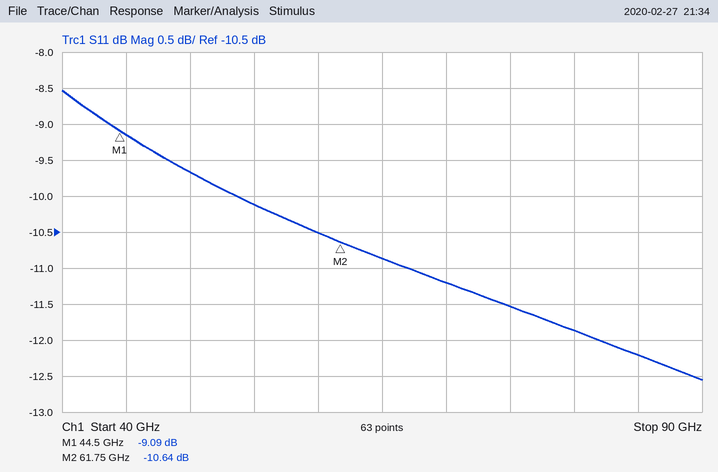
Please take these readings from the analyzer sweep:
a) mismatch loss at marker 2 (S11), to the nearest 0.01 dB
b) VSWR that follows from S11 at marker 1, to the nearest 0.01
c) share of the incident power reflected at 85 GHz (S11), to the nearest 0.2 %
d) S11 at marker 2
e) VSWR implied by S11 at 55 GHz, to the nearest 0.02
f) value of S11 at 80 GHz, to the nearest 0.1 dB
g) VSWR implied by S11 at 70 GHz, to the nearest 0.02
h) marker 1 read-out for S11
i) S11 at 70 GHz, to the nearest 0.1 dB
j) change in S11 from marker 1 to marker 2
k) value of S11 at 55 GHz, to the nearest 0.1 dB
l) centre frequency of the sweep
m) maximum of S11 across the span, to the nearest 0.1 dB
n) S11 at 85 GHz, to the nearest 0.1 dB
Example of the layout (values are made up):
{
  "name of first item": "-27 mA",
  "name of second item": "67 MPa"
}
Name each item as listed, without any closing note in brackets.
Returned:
{
  "mismatch loss at marker 2 (S11), to the nearest 0.01 dB": "0.39 dB",
  "VSWR that follows from S11 at marker 1, to the nearest 0.01": "2.08",
  "share of the incident power reflected at 85 GHz (S11), to the nearest 0.2 %": "6.0 %",
  "S11 at marker 2": "-10.64 dB",
  "VSWR implied by S11 at 55 GHz, to the nearest 0.02": "1.90",
  "value of S11 at 80 GHz, to the nearest 0.1 dB": "-11.9 dB",
  "VSWR implied by S11 at 70 GHz, to the nearest 0.02": "1.76",
  "marker 1 read-out for S11": "-9.09 dB",
  "S11 at 70 GHz, to the nearest 0.1 dB": "-11.2 dB",
  "change in S11 from marker 1 to marker 2": "-1.55 dB",
  "value of S11 at 55 GHz, to the nearest 0.1 dB": "-10.1 dB",
  "centre frequency of the sweep": "65 GHz",
  "maximum of S11 across the span, to the nearest 0.1 dB": "-8.5 dB",
  "S11 at 85 GHz, to the nearest 0.1 dB": "-12.2 dB"
}
